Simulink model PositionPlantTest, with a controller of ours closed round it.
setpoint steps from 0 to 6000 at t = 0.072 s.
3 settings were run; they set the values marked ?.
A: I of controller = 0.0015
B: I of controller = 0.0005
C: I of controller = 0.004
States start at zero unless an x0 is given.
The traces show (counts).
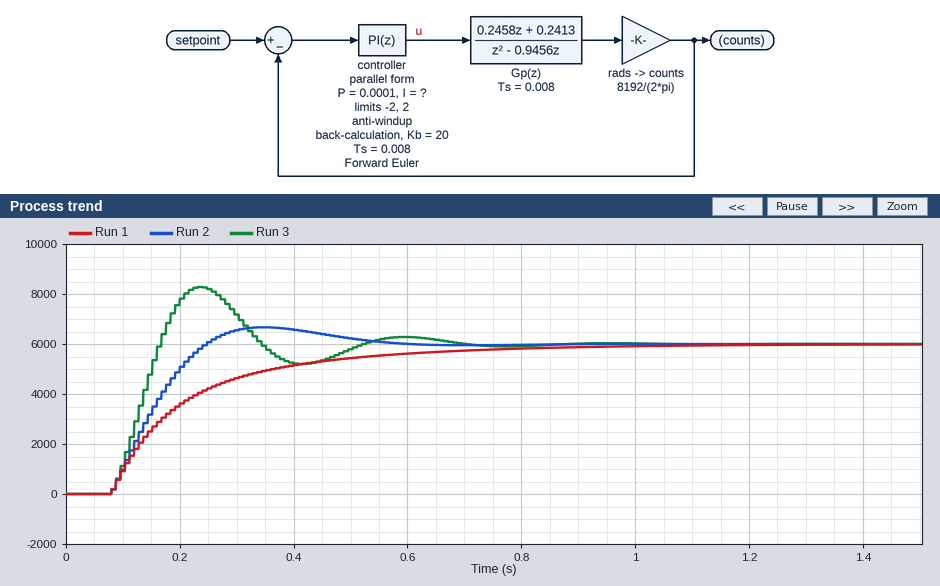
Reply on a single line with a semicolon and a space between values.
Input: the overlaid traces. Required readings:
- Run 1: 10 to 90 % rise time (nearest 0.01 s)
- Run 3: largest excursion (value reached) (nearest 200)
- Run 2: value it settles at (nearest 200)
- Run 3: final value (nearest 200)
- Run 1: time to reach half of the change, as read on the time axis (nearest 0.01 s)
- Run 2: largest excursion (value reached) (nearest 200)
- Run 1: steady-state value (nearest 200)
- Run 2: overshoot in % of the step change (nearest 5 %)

0.39 s; 8200; 6000; 6000; 0.17 s; 6600; 6000; 10 %
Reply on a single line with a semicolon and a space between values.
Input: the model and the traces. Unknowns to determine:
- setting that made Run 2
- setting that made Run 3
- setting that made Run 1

A; C; B
